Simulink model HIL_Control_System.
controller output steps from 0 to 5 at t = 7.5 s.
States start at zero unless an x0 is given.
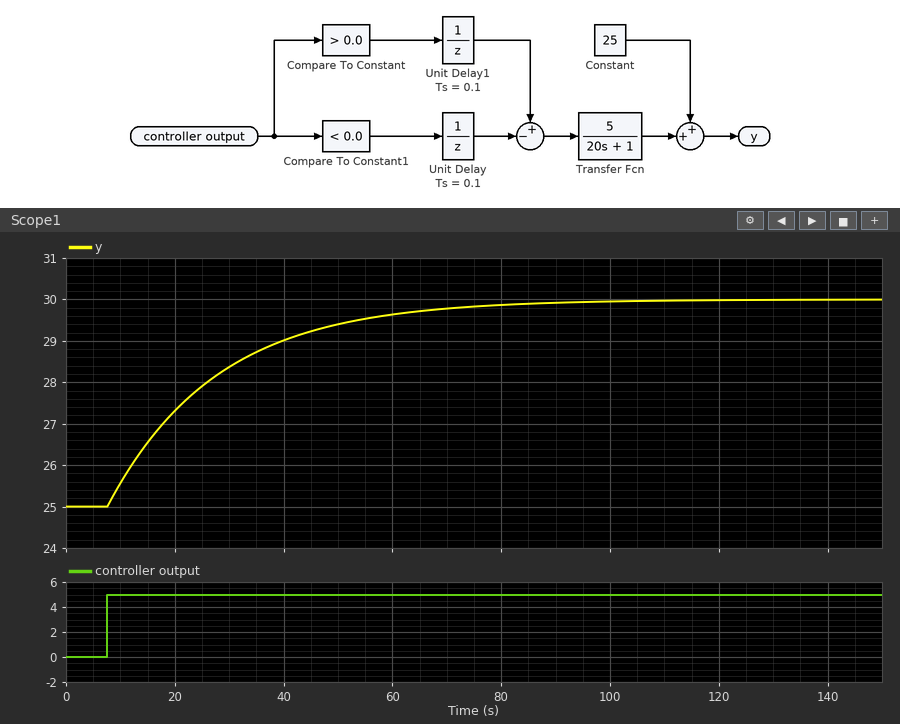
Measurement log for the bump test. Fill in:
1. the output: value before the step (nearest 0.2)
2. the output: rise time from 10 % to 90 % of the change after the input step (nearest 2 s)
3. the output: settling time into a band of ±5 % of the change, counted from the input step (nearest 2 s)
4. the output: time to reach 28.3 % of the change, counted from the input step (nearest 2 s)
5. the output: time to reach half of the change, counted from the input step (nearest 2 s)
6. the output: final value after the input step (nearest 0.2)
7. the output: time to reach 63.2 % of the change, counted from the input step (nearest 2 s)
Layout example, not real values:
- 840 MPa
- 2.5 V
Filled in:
- 25.0
- 44 s
- 60 s
- 6 s
- 14 s
- 30.0
- 20 s
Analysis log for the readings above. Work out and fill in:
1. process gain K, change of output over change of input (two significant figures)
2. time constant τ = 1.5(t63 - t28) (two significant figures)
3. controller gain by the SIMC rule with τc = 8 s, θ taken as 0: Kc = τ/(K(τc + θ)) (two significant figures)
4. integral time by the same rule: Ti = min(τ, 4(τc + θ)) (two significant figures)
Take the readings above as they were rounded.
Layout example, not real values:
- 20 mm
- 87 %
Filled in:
- 1.0
- 21 s
- 2.6
- 21 s
